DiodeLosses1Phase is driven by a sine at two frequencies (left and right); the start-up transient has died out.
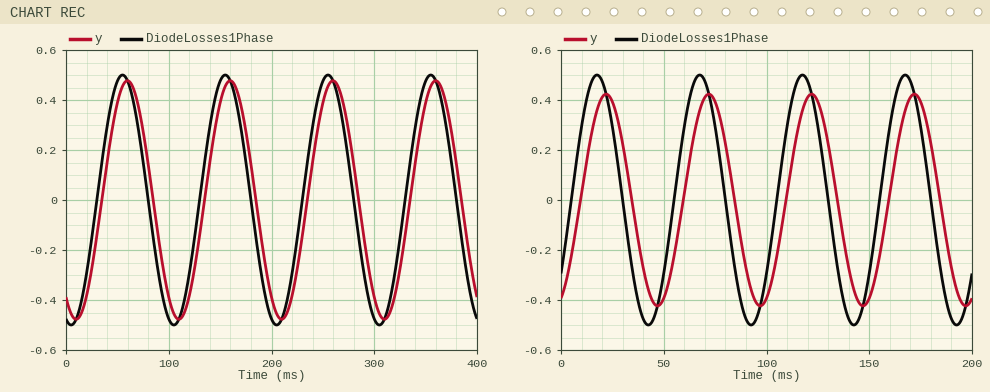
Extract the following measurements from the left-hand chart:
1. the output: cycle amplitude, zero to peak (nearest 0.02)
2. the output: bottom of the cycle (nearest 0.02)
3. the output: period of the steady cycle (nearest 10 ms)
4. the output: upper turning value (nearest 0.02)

0.48
-0.48
100 ms
0.48
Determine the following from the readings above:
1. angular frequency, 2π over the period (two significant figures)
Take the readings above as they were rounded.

0.063 rad/ms
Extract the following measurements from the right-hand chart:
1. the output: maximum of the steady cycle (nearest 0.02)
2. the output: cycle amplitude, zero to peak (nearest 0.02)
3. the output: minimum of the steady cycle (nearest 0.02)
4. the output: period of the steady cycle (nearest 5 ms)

0.42
0.42
-0.42
50 ms
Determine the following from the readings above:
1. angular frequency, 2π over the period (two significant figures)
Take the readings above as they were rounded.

0.13 rad/ms
